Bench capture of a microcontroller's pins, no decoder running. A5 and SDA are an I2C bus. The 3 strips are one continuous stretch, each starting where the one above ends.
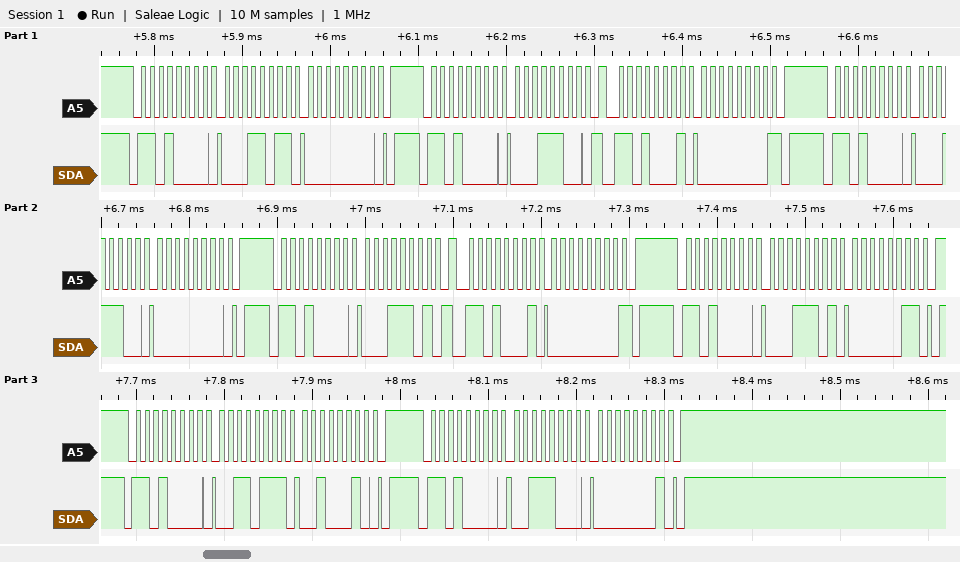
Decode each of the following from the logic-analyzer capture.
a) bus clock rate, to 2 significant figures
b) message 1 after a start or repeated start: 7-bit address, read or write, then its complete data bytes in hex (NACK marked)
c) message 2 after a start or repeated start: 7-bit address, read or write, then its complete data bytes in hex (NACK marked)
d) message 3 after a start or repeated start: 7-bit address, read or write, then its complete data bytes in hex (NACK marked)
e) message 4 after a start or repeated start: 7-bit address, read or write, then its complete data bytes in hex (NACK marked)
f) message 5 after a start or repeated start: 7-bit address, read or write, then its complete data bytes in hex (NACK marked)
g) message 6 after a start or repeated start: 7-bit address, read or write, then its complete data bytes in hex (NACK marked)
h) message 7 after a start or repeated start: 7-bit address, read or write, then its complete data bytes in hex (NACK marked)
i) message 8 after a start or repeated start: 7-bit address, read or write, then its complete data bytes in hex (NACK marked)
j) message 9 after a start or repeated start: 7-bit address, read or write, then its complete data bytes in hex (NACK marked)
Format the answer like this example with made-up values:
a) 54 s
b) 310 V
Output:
a) 100 kHz
b) 0x68 write: 1B 00
c) 0x68 write: 1C
d) 0x68 read: 00 NACK
e) 0x68 write: 1C 00
f) 0x68 write: 1D
g) 0x68 read: 00 NACK
h) 0x68 write: 1D 03
i) 0x68 write: 37 22
j) 0x68 write: 38 01
